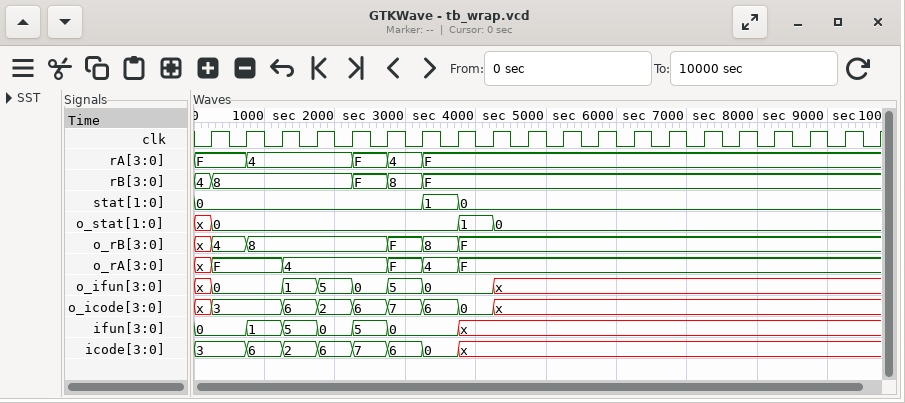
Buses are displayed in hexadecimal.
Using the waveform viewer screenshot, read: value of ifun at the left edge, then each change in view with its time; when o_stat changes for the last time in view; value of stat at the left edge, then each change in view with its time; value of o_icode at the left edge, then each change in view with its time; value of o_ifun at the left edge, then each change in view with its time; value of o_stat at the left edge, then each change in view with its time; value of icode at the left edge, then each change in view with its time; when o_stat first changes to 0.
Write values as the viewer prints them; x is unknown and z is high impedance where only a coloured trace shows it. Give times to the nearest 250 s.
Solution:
0, 1 at 750 s, 5 at 1250 s, 0 at 1750 s, 5 at 2250 s, 0 at 2750 s, x at 3750 s
4250 s
0, 1 at 3250 s, 0 at 3750 s
x, 3 at 250 s, 6 at 1250 s, 2 at 1750 s, 6 at 2250 s, 7 at 2750 s, 6 at 3250 s, 0 at 3750 s, x at 4250 s
x, 0 at 250 s, 1 at 1250 s, 5 at 1750 s, 0 at 2250 s, 5 at 2750 s, 0 at 3250 s, x at 4250 s
x, 0 at 250 s, 1 at 3750 s, 0 at 4250 s
3, 6 at 750 s, 2 at 1250 s, 6 at 1750 s, 7 at 2250 s, 6 at 2750 s, 0 at 3250 s, x at 3750 s
250 s
